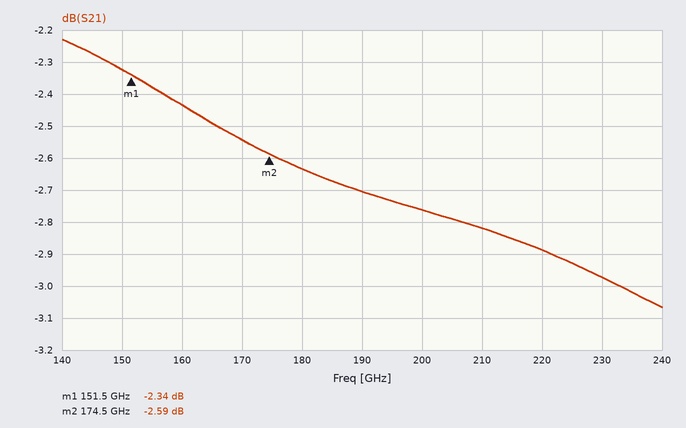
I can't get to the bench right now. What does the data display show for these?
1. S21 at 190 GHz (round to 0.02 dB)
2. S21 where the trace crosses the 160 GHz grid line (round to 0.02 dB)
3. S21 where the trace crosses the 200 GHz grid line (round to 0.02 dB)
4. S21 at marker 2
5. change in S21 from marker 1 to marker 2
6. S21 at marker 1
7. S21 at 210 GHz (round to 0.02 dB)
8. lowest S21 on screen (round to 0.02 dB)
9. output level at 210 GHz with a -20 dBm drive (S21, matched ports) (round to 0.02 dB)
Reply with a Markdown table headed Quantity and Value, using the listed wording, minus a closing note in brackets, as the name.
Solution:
| Quantity | Value |
|---|---|
| S21 at 190 GHz | -2.70 dB |
| S21 where the trace crosses the 160 GHz grid line | -2.44 dB |
| S21 where the trace crosses the 200 GHz grid line | -2.76 dB |
| S21 at marker 2 | -2.59 dB |
| change in S21 from marker 1 to marker 2 | -0.25 dB |
| S21 at marker 1 | -2.34 dB |
| S21 at 210 GHz | -2.82 dB |
| lowest S21 on screen | -3.06 dB |
| output level at 210 GHz with a -20 dBm drive (S21, matched ports) | -22.82 dBm |
